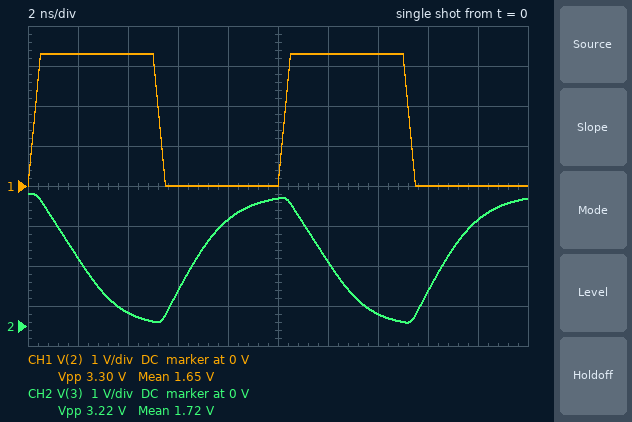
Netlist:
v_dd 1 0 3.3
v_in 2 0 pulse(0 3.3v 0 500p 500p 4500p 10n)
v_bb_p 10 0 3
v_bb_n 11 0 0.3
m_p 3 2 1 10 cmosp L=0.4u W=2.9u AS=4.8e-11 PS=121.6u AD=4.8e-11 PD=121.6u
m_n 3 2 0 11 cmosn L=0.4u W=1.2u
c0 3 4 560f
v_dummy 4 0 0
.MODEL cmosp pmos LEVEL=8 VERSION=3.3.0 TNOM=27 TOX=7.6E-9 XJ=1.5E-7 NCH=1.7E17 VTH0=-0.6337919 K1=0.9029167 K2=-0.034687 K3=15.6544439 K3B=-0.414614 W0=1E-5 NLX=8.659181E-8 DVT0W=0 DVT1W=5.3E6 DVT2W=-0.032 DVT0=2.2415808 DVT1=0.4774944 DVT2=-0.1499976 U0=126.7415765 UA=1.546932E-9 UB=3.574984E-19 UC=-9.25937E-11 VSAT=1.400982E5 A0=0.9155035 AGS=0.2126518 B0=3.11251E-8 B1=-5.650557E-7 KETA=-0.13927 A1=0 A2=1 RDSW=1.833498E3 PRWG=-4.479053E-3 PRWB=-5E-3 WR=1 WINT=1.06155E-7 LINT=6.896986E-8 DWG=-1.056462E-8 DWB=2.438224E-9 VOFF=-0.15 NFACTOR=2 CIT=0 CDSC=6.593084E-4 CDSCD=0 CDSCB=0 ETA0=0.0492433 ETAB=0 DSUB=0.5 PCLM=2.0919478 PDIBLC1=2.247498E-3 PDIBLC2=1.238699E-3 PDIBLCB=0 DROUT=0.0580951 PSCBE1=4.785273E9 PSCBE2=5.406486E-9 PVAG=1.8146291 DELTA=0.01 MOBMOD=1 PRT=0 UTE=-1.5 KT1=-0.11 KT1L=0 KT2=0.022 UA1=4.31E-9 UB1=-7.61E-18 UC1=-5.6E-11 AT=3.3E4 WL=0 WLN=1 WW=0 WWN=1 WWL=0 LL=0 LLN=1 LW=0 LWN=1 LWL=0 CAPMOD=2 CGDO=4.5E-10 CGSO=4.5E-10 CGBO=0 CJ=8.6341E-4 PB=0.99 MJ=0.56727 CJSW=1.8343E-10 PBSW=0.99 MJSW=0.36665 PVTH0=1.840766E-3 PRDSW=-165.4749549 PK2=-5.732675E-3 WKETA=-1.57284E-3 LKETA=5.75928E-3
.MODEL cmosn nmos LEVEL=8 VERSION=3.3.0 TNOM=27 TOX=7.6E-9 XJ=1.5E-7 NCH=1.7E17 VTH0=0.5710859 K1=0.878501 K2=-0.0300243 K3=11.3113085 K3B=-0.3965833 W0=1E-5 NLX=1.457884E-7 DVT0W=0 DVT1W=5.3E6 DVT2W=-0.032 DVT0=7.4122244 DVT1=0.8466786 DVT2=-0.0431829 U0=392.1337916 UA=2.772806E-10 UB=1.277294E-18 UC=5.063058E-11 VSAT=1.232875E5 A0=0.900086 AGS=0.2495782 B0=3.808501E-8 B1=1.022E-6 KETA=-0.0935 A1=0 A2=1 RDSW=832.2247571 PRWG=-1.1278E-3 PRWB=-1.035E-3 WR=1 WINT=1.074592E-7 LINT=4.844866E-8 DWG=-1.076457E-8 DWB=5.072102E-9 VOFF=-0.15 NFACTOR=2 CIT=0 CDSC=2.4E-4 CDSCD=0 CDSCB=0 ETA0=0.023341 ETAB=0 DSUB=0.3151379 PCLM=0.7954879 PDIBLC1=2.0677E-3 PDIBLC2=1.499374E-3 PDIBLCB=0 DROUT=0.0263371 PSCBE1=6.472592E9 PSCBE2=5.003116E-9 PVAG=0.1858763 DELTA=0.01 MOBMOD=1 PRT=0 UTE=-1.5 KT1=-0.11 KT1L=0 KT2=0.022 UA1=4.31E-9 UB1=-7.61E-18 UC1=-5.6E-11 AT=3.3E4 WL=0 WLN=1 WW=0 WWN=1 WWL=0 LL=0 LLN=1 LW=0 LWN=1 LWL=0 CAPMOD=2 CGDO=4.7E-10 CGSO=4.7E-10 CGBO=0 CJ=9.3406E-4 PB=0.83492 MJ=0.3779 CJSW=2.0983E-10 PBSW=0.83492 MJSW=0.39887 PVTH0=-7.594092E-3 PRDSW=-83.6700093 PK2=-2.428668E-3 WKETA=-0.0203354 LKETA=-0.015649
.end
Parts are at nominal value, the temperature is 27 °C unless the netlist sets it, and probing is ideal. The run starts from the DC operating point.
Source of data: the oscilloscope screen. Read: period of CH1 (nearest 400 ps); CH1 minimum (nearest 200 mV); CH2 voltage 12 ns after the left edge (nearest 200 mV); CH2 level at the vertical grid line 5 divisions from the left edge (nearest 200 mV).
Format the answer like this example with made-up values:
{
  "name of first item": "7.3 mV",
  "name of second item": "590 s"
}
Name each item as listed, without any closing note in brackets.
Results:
{
  "period of CH1": "10.0 ns",
  "CH1 minimum": "0 V",
  "CH2 voltage 12 ns after the left edge": "1.6 V",
  "CH2 level at the vertical grid line 5 divisions from the left edge": "3.2 V"
}
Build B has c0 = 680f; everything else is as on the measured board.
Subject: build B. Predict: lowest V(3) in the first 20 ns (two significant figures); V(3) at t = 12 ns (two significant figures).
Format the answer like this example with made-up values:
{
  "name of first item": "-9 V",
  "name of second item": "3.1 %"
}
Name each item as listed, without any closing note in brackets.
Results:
{
  "lowest V(3) in the first 20 ns": "180 mV",
  "V(3) at t = 12 ns": "1.8 V"
}
